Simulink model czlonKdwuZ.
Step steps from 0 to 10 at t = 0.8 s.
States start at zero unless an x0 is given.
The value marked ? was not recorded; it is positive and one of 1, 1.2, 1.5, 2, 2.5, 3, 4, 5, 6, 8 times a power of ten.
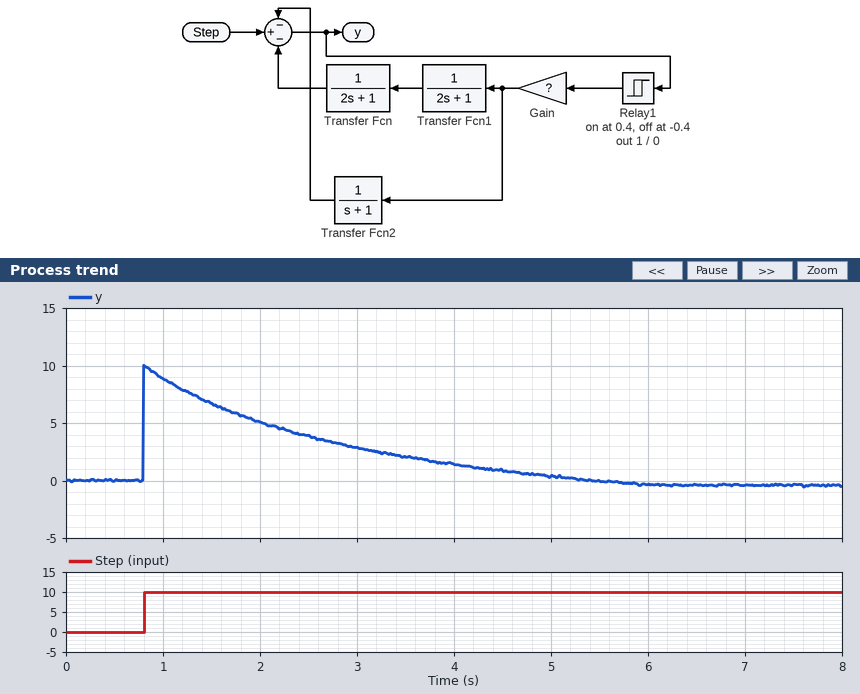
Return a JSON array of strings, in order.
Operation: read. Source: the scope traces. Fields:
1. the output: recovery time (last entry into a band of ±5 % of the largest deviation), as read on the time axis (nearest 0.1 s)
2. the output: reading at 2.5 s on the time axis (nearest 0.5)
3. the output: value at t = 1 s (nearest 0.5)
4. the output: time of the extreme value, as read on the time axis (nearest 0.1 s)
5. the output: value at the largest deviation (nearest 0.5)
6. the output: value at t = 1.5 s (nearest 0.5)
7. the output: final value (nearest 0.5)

["5.3 s", "4.0", "9.0", "0.8 s", "10.0", "6.5", "-0.5"]
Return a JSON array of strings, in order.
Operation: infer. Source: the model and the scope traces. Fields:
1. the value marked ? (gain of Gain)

["6"]
